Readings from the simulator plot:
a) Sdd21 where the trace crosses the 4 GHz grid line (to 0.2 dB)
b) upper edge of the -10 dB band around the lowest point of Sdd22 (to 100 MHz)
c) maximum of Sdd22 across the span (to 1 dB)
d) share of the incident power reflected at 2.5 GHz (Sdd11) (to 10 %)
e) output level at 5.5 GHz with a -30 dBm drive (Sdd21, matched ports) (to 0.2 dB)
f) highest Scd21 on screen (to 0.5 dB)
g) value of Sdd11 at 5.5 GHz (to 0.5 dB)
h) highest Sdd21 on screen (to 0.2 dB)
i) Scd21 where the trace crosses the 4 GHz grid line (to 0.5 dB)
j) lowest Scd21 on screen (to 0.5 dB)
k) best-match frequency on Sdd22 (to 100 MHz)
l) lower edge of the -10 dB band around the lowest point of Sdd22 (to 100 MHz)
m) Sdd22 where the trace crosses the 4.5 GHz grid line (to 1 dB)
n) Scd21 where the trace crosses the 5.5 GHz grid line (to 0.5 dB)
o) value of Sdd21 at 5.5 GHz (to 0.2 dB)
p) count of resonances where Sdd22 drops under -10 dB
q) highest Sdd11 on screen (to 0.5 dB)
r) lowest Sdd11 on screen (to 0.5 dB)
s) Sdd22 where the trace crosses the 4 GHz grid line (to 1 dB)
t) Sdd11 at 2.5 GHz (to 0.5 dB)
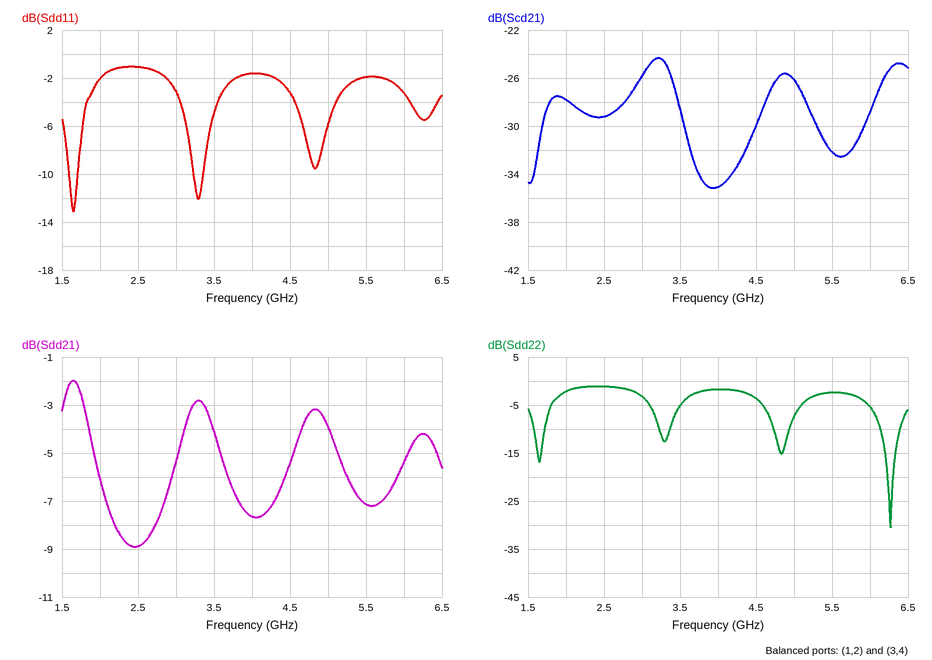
-7.6 dB
6.4 GHz
-1 dB
80 %
-37.2 dBm
-24.5 dB
-2.0 dB
-2.0 dB
-35.0 dB
-35.0 dB
6.3 GHz
6.1 GHz
-4 dB
-32.0 dB
-7.2 dB
4
-1.0 dB
-13.0 dB
-2 dB
-1.0 dB
